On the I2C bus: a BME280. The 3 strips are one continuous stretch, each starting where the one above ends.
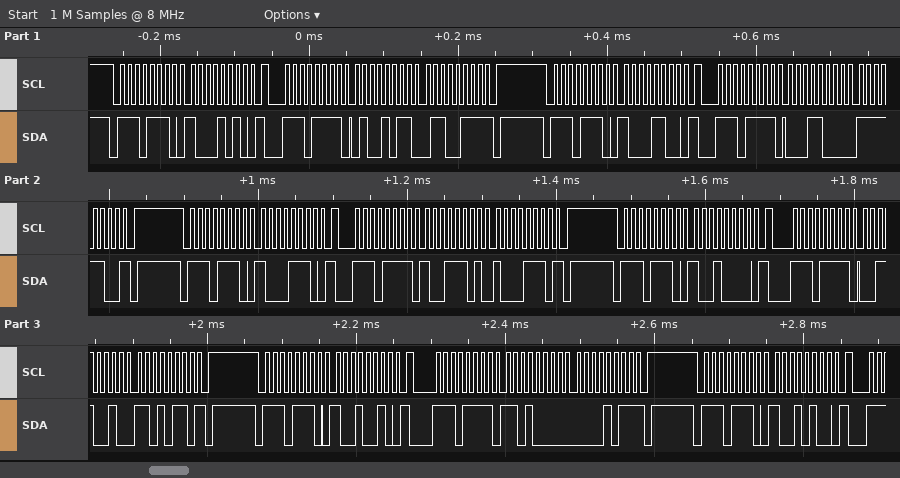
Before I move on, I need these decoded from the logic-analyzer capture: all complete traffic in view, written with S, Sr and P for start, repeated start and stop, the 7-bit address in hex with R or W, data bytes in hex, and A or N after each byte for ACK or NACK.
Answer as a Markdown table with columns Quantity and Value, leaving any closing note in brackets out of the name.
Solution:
| Quantity | Value |
|---|---|
| all complete traffic in view, written with S, Sr and P for start, repeated start and stop, the 7-bit address in hex with R or W, data bytes in hex, and A or N after each byte for ACK or NACK | S 77W A 8A A Sr 77R A 4B A 67 N P S 77W A 8C A Sr 77R A 18 A FC N P S 77W A 8E A Sr 77R A 9D A 8E N P S 77W A 90 A Sr 77R A 32 A D6 N P S 77W A 92 A Sr 77R A D0 A 0B N P S 77W A 94 A |
